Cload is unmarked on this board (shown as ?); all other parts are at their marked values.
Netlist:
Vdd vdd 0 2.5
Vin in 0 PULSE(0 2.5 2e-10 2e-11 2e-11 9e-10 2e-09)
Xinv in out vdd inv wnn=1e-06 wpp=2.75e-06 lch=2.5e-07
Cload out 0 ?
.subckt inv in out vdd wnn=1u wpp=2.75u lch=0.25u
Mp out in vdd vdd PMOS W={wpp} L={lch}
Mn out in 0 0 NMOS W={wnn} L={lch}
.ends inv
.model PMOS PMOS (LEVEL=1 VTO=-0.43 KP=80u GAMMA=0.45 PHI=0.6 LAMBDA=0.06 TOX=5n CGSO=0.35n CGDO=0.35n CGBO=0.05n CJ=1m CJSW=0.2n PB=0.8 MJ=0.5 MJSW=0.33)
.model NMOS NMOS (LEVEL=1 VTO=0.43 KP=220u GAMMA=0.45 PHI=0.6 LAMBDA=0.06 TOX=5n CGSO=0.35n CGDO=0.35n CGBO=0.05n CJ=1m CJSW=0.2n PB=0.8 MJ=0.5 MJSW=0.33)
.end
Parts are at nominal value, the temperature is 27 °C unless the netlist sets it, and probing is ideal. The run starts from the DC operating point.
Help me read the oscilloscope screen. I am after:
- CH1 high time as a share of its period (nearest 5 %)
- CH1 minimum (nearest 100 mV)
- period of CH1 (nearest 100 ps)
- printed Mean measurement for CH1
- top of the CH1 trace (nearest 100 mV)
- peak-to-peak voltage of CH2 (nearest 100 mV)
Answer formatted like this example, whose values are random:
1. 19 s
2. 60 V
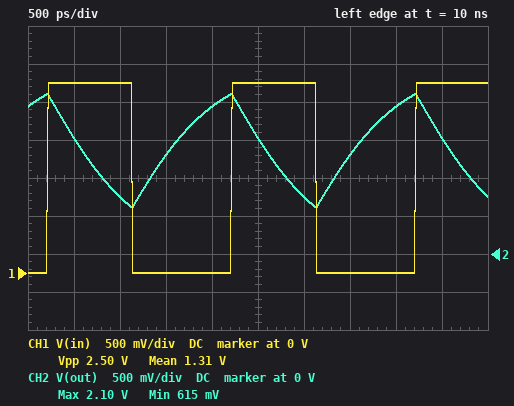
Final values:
1. 45 %
2. 0 V
3. 2.0 ns
4. 1.31 V
5. 2.5 V
6. 1.5 V
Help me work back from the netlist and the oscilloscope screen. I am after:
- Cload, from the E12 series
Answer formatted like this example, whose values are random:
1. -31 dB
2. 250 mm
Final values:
1. 1 pF
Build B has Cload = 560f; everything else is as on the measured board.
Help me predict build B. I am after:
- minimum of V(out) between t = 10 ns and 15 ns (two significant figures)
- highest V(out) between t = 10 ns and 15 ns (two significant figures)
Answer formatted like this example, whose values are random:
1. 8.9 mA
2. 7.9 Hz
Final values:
1. 230 mV
2. 2.4 V
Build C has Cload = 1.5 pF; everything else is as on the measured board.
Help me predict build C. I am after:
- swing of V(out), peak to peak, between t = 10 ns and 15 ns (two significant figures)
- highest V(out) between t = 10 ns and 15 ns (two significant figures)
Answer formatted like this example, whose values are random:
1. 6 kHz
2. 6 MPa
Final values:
1. 1.1 V
2. 1.9 V
